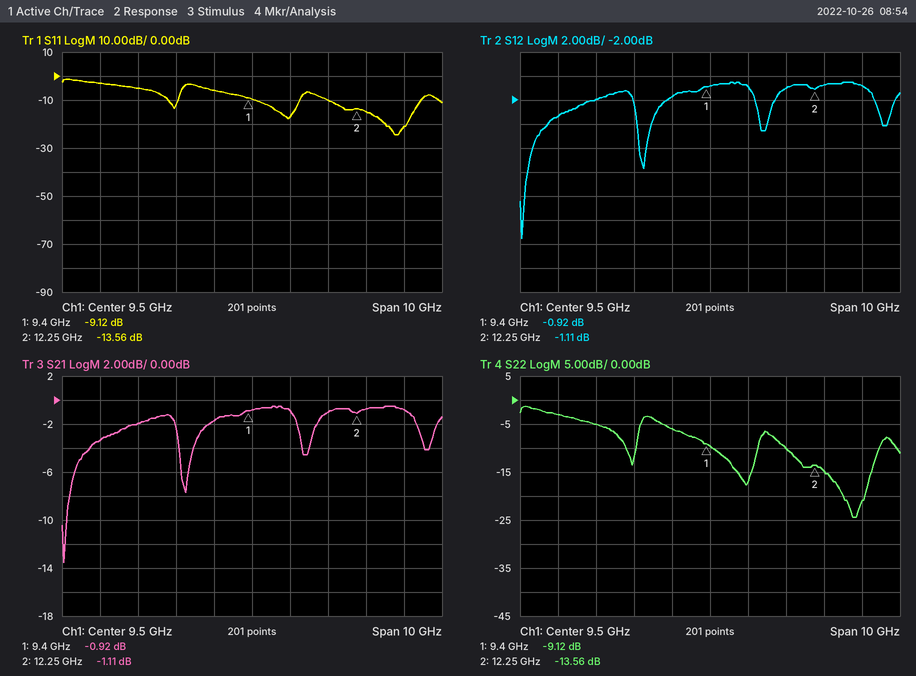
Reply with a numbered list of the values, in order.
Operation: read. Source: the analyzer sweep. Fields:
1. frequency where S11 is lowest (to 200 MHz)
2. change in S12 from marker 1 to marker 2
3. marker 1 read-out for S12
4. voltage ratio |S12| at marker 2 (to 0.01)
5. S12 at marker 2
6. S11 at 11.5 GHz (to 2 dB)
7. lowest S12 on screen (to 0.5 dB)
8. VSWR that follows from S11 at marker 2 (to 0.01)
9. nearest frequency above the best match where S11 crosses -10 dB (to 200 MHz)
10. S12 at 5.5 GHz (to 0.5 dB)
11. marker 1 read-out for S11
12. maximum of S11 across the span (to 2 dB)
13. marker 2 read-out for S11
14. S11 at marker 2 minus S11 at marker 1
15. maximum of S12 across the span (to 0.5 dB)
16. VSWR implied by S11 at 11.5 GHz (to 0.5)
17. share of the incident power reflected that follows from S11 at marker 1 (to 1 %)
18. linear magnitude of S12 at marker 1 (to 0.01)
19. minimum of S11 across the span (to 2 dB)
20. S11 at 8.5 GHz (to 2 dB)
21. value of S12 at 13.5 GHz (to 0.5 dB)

1. 13.2 GHz
2. -0.19 dB
3. -0.92 dB
4. 0.88
5. -1.11 dB
6. -10 dB
7. -13.5 dB
8. 1.53
9. 14.0 GHz
10. -3.5 dB
11. -9.12 dB
12. -2 dB
13. -13.56 dB
14. -4.44 dB
15. -0.5 dB
16. 2.0
17. 12 %
18. 0.90
19. -24 dB
20. -6 dB
21. -1.0 dB
